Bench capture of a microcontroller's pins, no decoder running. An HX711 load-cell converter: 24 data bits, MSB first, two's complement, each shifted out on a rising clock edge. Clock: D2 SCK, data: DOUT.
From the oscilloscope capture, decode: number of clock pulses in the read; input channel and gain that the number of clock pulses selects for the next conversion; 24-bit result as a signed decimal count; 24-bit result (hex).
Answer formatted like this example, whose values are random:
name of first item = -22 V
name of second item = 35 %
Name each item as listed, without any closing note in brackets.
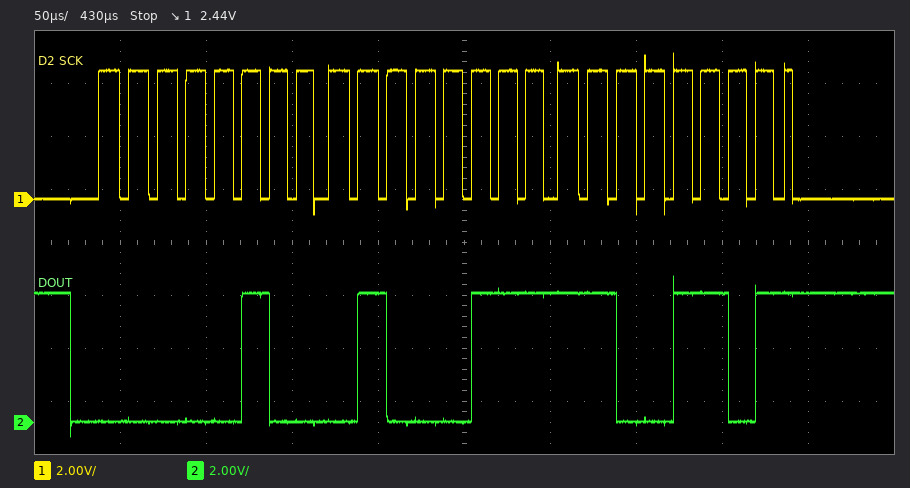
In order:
number of clock pulses in the read = 25
input channel and gain that the number of clock pulses selects for the next conversion = channel A, gain 128
24-bit result as a signed decimal count = 280525
24-bit result = 0x0447CD
